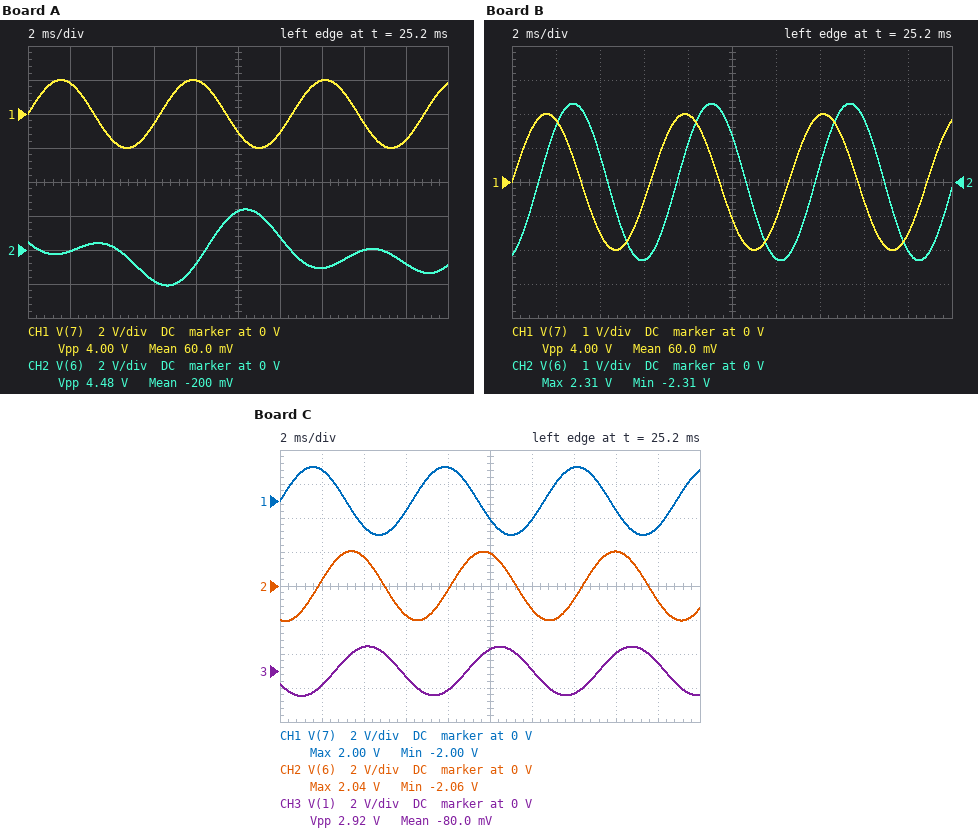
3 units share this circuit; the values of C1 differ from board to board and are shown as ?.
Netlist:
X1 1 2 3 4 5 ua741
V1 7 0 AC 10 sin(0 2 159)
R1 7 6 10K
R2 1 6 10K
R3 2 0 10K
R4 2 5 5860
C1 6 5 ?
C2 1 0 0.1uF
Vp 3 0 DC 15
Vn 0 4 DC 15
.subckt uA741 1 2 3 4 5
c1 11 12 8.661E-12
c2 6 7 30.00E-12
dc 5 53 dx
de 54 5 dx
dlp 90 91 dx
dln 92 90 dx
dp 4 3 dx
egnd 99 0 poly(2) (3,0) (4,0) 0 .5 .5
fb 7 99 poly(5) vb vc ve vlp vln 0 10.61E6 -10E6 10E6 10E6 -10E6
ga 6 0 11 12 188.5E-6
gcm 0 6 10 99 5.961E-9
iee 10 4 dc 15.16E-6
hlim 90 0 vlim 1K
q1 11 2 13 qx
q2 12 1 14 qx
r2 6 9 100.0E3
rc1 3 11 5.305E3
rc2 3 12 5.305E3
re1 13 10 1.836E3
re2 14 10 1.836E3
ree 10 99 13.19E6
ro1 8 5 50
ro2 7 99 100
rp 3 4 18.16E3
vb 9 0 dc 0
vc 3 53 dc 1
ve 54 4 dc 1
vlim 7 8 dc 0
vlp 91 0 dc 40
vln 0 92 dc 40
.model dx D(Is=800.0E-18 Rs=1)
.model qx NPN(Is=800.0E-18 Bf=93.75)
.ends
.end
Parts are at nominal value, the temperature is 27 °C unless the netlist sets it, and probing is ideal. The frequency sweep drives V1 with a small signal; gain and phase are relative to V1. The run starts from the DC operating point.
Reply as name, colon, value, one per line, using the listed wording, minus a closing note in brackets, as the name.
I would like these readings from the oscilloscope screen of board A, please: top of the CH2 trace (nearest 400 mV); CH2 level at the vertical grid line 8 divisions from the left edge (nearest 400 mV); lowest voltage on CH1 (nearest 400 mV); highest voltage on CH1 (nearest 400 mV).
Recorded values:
top of the CH2 trace: 2.4 V
CH2 level at the vertical grid line 8 divisions from the left edge: 0 V
lowest voltage on CH1: -2.0 V
highest voltage on CH1: 2.0 V
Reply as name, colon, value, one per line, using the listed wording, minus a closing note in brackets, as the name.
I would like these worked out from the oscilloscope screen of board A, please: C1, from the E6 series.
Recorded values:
C1, from the E6 series: 330 nF
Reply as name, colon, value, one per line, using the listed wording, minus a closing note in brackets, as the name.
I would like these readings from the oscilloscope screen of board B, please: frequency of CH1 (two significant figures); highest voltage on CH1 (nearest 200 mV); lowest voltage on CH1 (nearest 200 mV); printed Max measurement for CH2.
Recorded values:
frequency of CH1: 160 Hz
highest voltage on CH1: 2.0 V
lowest voltage on CH1: -2.0 V
printed Max measurement for CH2: 2.31 V
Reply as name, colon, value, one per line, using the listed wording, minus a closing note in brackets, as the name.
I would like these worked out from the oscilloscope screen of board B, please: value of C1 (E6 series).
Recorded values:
value of C1: 150 nF
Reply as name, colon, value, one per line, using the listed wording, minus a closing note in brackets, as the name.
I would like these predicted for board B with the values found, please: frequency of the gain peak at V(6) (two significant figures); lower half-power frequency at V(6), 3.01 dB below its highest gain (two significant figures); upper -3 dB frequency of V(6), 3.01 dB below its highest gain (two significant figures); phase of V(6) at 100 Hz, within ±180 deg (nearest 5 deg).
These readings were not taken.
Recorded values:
frequency of the gain peak at V(6): 110 Hz
lower half-power frequency at V(6), 3.01 dB below its highest gain: 28 Hz
upper -3 dB frequency of V(6), 3.01 dB below its highest gain: 170 Hz
phase of V(6) at 100 Hz, within ±180 deg: -30 deg
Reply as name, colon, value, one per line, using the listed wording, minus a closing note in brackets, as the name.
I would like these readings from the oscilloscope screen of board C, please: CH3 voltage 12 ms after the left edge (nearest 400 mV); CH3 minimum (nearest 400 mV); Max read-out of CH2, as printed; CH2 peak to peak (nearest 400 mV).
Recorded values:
CH3 voltage 12 ms after the left edge: 0 V
CH3 minimum: -1.6 V
Max read-out of CH2, as printed: 2.04 V
CH2 peak to peak: 4.0 V
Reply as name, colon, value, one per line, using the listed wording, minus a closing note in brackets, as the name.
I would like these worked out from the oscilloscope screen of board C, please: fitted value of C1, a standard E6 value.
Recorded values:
fitted value of C1, a standard E6 value: 220 nF
